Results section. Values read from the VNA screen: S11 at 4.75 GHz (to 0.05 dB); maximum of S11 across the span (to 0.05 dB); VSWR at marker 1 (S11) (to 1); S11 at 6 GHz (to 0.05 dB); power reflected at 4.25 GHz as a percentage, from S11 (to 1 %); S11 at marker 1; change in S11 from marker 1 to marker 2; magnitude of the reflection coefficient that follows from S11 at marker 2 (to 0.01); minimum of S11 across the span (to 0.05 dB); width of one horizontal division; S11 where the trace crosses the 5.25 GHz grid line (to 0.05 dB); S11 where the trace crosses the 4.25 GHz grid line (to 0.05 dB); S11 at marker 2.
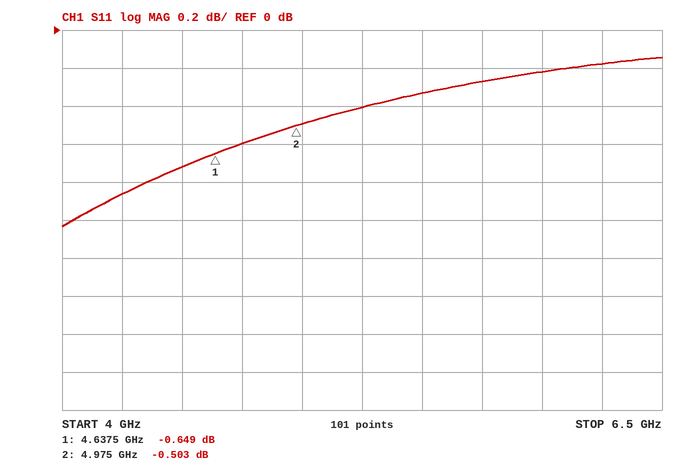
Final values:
-0.60 dB
-0.15 dB
27
-0.20 dB
82 %
-0.649 dB
0.146 dB
0.94
-1.05 dB
250 MHz
-0.40 dB
-0.85 dB
-0.503 dB
